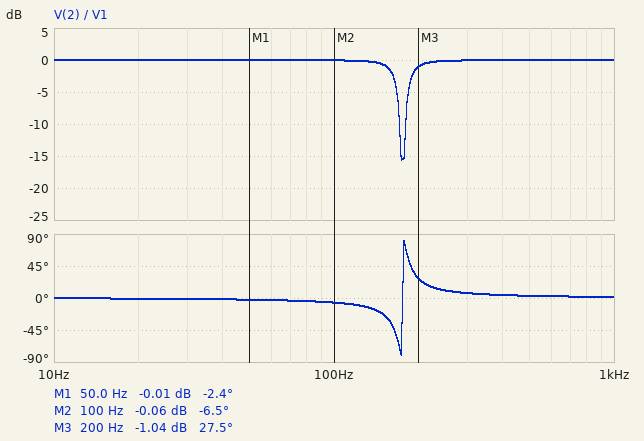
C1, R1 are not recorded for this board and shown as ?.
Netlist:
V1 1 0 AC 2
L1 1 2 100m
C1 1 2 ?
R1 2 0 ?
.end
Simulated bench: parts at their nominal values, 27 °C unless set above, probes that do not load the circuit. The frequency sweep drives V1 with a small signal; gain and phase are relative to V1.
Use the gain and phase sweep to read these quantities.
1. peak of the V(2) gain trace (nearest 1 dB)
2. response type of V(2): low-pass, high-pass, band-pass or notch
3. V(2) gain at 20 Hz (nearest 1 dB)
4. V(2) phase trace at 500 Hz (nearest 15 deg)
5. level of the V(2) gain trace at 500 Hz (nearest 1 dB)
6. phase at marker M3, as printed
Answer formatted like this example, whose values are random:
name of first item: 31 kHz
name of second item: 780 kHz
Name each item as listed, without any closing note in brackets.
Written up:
peak of the V(2) gain trace: 0 dB
response type of V(2): low-pass, high-pass, band-pass or notch: notch
V(2) gain at 20 Hz: 0 dB
V(2) phase trace at 500 Hz: 0 deg
level of the V(2) gain trace at 500 Hz: 0 dB
phase at marker M3, as printed: 27.5 deg
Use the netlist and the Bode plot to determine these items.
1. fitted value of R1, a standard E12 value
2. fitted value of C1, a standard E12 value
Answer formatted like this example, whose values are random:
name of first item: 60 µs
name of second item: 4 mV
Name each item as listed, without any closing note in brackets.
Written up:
fitted value of R1, a standard E12 value: 820 Ω
fitted value of C1, a standard E12 value: 8.2 µF
